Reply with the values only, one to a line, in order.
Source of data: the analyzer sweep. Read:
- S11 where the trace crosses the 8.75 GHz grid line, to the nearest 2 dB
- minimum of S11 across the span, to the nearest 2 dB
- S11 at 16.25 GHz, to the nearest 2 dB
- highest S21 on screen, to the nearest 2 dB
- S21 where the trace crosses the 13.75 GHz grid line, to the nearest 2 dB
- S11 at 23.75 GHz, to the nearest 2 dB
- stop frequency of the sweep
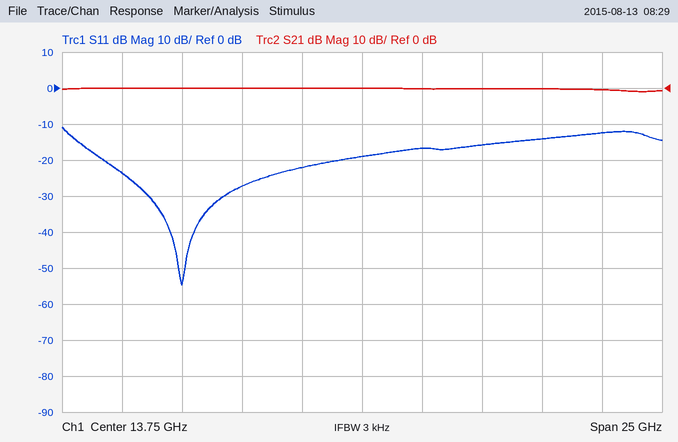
-28 dB
-54 dB
-16 dB
0 dB
0 dB
-12 dB
26.25 GHz
